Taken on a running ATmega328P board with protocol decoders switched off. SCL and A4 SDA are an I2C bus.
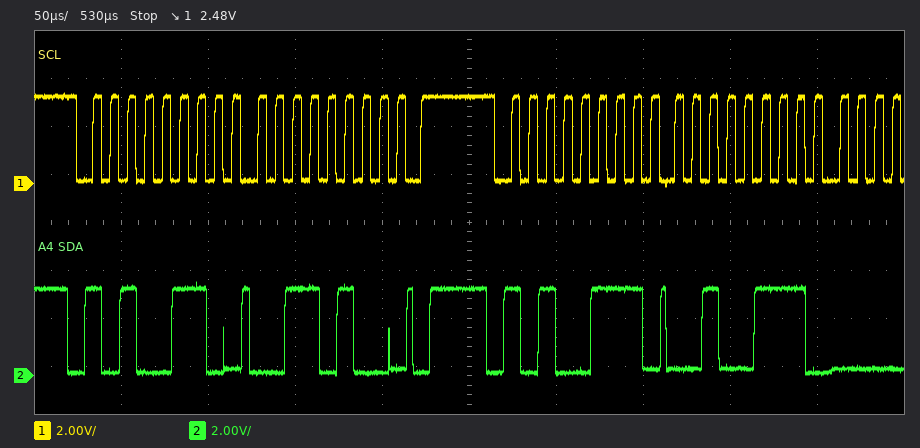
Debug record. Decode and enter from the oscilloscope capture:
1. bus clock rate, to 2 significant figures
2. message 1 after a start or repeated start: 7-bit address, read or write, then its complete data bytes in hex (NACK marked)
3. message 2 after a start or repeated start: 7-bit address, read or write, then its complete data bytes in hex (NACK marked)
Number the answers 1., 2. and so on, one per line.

1. 100 kHz
2. 0x53 write: 34
3. 0x53 read: 27
